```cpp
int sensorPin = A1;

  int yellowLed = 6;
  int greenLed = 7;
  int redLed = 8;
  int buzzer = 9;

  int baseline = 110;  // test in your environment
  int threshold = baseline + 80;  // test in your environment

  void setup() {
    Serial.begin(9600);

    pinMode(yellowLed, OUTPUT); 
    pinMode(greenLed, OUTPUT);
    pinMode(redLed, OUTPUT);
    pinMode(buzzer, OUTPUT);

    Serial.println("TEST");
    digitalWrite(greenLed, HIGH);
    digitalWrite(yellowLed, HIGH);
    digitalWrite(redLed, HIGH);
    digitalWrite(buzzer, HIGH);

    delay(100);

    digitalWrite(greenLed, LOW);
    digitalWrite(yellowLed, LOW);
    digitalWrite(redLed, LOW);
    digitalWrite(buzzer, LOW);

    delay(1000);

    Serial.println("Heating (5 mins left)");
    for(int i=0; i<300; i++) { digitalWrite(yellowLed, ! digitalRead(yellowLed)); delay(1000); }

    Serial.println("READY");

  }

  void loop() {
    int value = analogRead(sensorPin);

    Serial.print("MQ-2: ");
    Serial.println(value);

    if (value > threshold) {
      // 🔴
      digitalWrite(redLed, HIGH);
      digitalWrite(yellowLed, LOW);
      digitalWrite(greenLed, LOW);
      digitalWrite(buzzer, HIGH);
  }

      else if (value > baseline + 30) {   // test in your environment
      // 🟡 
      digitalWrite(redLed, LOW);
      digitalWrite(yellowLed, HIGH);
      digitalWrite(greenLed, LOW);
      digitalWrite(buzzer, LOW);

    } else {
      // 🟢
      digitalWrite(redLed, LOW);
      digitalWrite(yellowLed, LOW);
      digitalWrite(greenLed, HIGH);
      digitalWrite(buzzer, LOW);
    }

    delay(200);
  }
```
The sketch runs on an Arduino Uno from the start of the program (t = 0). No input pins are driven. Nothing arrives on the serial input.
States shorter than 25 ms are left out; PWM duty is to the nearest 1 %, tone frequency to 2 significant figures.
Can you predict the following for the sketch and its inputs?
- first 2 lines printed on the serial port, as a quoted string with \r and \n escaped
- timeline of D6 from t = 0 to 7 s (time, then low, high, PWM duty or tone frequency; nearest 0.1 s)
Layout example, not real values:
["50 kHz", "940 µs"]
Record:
["\"TEST\\r\\nHeating (5 mins left)\\r\\n\"", "0 s high; 0.1 s low; 1.1 s high; 2.1 s low; 3.1 s high; 4.1 s low; 5.1 s high; 6.1 s low"]
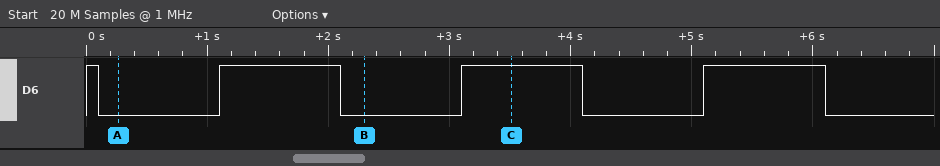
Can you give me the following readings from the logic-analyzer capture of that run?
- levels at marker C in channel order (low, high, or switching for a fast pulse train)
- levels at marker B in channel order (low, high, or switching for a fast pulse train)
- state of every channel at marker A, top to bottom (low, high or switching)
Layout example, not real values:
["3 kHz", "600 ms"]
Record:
["D6 high", "D6 low", "D6 low"]
